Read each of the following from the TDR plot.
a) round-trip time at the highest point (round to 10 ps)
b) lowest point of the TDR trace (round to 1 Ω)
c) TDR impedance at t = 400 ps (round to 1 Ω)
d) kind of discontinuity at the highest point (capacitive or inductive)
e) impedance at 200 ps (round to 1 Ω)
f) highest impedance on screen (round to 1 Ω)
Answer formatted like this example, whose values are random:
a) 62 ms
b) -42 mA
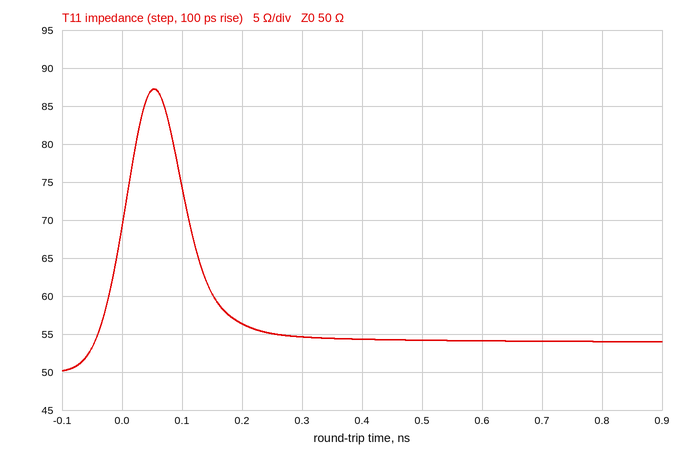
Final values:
a) 50 ps
b) 50 Ω
c) 54 Ω
d) inductive
e) 56 Ω
f) 87 Ω
